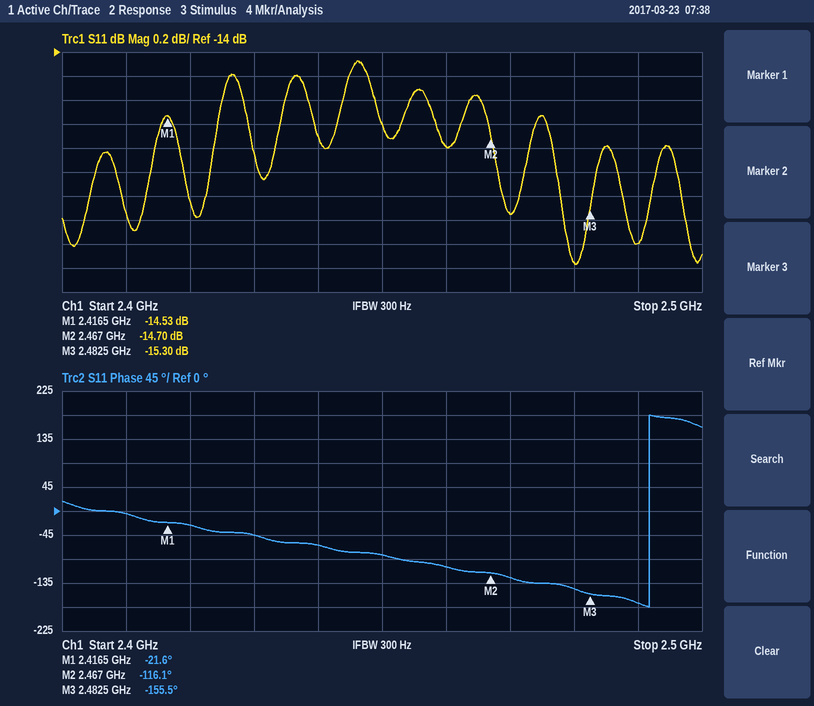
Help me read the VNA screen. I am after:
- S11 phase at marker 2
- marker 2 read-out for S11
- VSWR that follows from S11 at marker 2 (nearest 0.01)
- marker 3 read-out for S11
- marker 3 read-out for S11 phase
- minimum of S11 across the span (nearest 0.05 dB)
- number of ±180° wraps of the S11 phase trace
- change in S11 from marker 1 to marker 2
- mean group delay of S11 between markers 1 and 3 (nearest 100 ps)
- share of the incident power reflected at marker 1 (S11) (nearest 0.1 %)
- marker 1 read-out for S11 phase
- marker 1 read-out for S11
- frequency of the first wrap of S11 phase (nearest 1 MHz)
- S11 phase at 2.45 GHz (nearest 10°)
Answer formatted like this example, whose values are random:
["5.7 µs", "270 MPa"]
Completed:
["-116.1°", "-14.70 dB", "1.45", "-15.30 dB", "-155.5°", "-15.75 dB", "1", "-0.17 dB", "5.6 ns", "3.5 %", "-21.6°", "-14.53 dB", "2.492 GHz", "-80°"]
